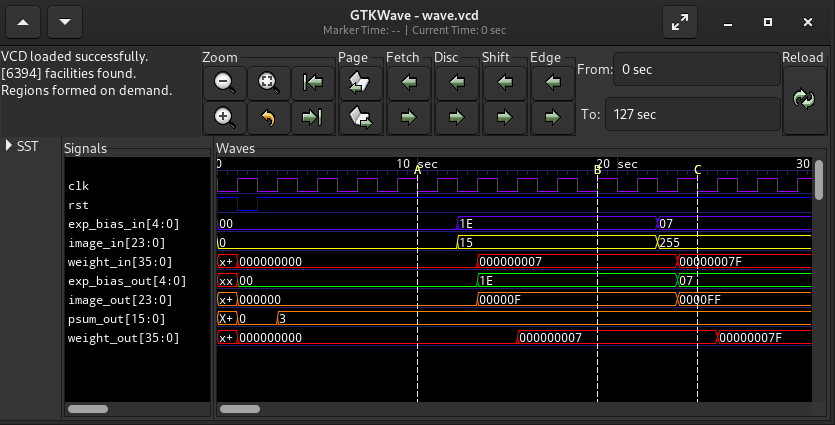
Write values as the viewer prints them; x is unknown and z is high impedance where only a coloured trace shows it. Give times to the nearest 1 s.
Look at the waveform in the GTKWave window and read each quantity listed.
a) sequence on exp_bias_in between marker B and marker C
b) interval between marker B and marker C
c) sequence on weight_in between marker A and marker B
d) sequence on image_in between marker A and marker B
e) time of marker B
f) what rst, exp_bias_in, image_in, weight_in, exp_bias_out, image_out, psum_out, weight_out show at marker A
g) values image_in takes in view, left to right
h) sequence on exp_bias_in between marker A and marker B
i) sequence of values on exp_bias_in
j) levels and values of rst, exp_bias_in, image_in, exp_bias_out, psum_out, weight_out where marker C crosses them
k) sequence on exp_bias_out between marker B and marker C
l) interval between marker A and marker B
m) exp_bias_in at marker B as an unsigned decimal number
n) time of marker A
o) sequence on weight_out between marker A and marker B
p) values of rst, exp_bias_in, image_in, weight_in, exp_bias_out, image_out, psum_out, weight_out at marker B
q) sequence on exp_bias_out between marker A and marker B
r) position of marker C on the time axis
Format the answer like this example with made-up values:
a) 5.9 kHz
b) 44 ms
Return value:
a) 1E, 07
b) 5 s
c) 000000000, 000000007
d) 0, 15
e) 19 s
f) rst=1, exp_bias_in=00, image_in=0, weight_in=000000000, exp_bias_out=00, image_out=000000, psum_out=3, weight_out=000000000
g) 0, 15, 255
h) 00, 1E
i) 00, 1E, 07
j) rst=1, exp_bias_in=07, image_in=255, exp_bias_out=07, psum_out=3, weight_out=000000007
k) 1E, 07
l) 9 s
m) 30
n) 10 s
o) 000000000, 000000007
p) rst=1, exp_bias_in=1E, image_in=15, weight_in=000000007, exp_bias_out=1E, image_out=00000F, psum_out=3, weight_out=000000007
q) 00, 1E
r) 24 s
